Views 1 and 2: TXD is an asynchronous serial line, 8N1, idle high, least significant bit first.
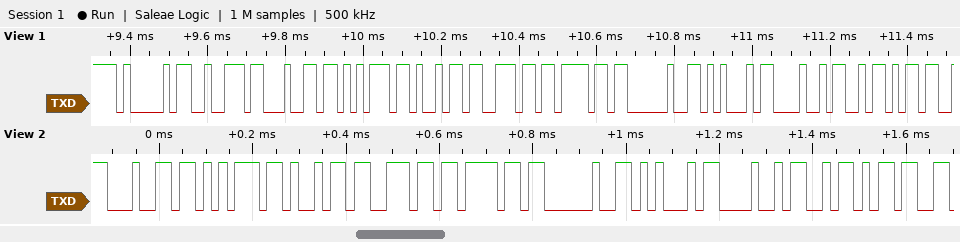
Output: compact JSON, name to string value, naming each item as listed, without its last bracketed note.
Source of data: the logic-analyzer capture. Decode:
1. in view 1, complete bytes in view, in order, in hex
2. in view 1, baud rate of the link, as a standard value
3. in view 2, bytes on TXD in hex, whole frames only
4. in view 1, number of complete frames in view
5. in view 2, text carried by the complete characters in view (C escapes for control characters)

{"in view 1, complete bytes in view, in order, in hex": "41 72 64 75 69 6E 6F 20 45 48 5A", "in view 1, baud rate of the link, as a standard value": "57600 baud", "in view 2, bytes on TXD in hex, whole frames only": "64 75 69 6E 6F 20 45 48 5A", "in view 1, number of complete frames in view": "11", "in view 2, text carried by the complete characters in view": "\"duino EHZ\""}
